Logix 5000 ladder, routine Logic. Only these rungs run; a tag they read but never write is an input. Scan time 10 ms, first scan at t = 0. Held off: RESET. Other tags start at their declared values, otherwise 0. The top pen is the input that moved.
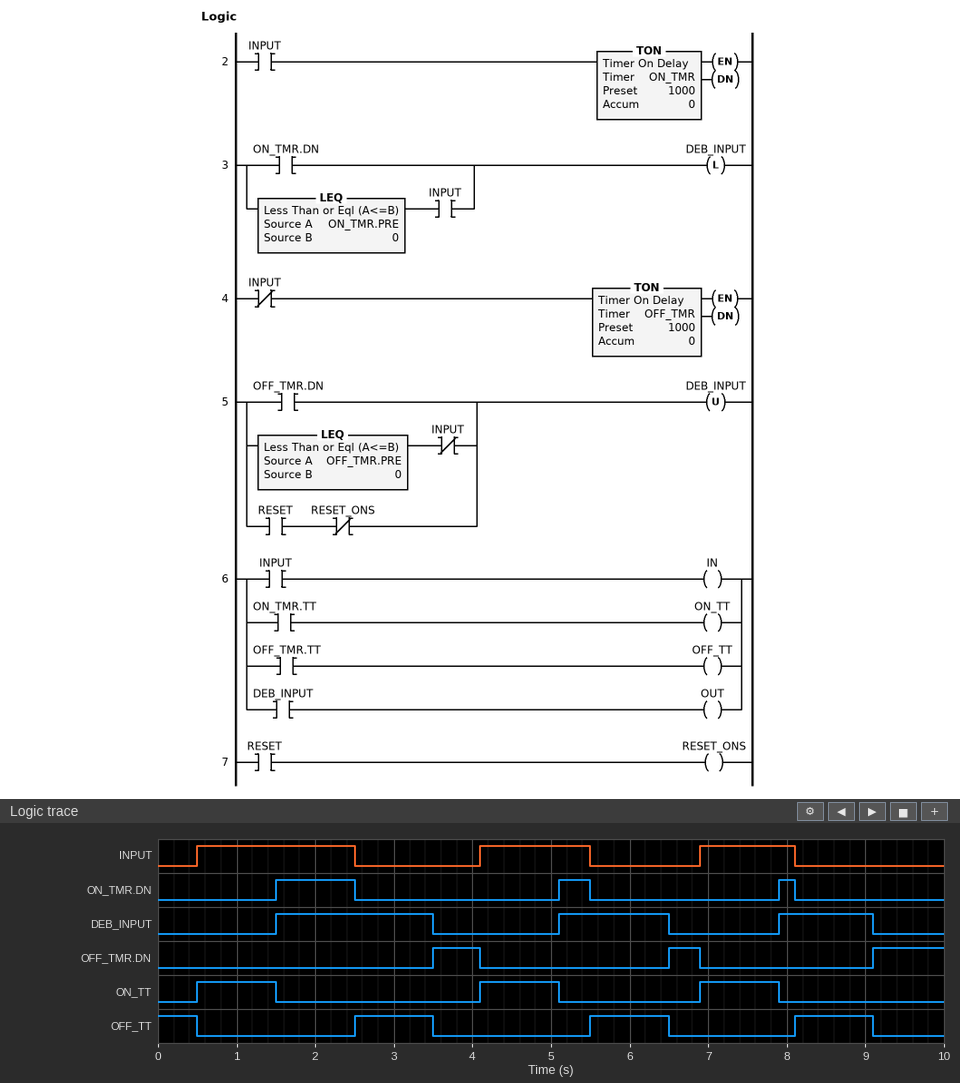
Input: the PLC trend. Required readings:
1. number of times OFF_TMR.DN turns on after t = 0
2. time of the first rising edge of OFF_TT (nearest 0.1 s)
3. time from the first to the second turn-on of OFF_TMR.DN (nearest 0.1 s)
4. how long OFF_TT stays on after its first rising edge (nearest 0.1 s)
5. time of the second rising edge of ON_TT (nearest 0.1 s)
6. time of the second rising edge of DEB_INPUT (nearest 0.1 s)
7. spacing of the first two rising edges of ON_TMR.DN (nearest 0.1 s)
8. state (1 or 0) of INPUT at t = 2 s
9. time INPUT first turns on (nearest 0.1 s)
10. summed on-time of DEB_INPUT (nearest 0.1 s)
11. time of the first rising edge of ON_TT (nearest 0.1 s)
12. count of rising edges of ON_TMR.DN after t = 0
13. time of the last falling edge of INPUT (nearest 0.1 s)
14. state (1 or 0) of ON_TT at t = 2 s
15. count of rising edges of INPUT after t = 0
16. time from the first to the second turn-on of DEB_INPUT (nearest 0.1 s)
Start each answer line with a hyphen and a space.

- 3
- 2.5 s
- 3.0 s
- 1.0 s
- 4.1 s
- 5.1 s
- 3.6 s
- 1
- 0.5 s
- 4.6 s
- 0.5 s
- 3
- 8.1 s
- 0
- 3
- 3.6 s
